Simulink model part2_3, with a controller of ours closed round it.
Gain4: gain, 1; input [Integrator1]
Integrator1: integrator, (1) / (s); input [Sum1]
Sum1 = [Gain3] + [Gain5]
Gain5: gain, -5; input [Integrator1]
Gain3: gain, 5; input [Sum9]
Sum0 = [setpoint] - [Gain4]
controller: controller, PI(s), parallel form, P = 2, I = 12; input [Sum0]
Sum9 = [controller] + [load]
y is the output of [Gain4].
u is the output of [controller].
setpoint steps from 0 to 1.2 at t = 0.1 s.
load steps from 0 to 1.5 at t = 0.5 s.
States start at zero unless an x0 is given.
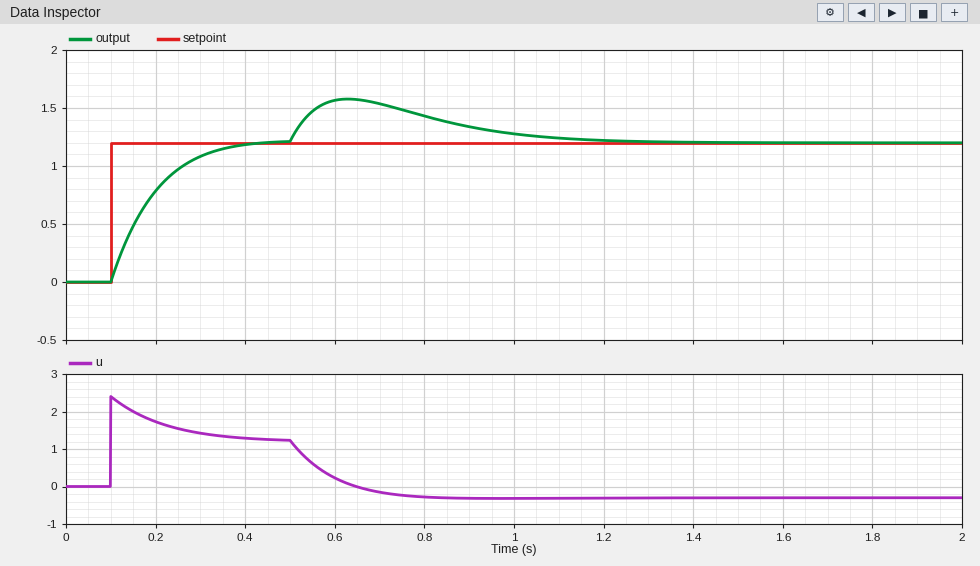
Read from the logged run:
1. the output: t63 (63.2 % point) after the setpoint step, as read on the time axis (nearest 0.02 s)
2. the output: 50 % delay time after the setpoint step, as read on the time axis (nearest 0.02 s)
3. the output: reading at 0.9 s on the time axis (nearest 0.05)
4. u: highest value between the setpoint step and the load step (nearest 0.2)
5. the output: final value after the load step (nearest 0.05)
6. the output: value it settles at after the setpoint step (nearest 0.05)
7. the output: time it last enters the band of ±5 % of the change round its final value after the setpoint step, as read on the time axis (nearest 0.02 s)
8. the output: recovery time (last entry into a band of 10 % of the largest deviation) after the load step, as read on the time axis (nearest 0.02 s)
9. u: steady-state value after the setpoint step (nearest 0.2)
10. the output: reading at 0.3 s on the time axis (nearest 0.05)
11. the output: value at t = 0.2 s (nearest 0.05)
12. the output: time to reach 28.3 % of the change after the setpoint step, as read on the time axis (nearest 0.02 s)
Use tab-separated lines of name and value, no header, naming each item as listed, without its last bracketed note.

the output: t63 (63.2 % point) after the setpoint step, as read on the time axis	0.20 s
the output: 50 % delay time after the setpoint step, as read on the time axis	0.16 s
the output: reading at 0.9 s on the time axis	1.35
u: highest value between the setpoint step and the load step	2.4
the output: final value after the load step	1.20
the output: value it settles at after the setpoint step	1.20
the output: time it last enters the band of ±5 % of the change round its final value after the setpoint step, as read on the time axis	0.34 s
the output: recovery time (last entry into a band of 10 % of the largest deviation) after the load step, as read on the time axis	1.12 s
u: steady-state value after the setpoint step	1.2
the output: reading at 0.3 s on the time axis	1.10
the output: value at t = 0.2 s	0.80
the output: time to reach 28.3 % of the change after the setpoint step, as read on the time axis	0.14 s
